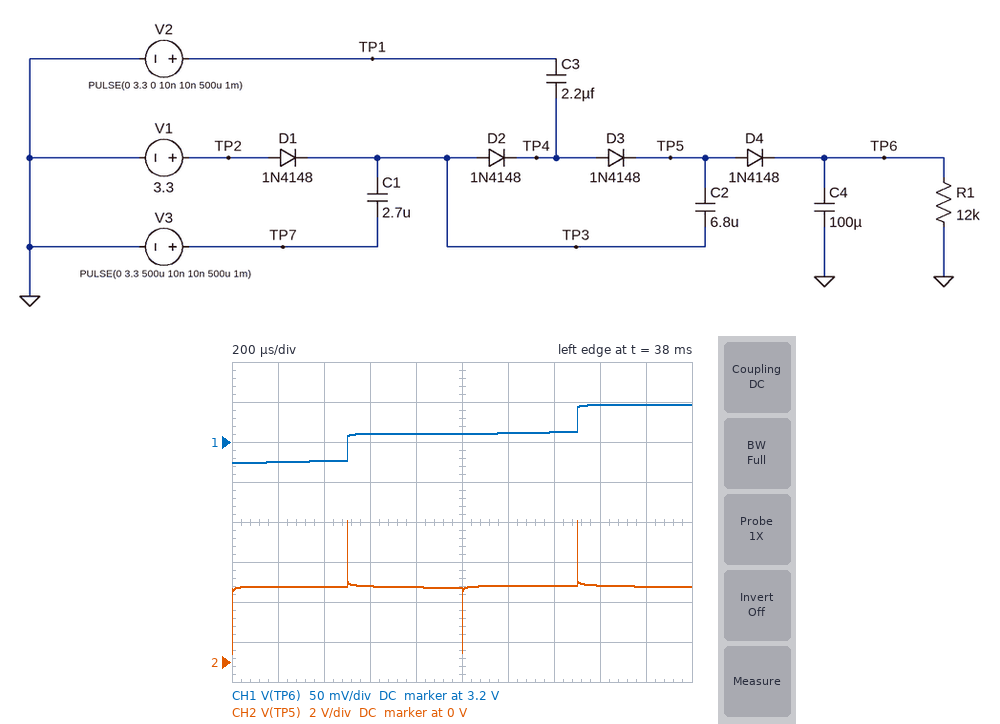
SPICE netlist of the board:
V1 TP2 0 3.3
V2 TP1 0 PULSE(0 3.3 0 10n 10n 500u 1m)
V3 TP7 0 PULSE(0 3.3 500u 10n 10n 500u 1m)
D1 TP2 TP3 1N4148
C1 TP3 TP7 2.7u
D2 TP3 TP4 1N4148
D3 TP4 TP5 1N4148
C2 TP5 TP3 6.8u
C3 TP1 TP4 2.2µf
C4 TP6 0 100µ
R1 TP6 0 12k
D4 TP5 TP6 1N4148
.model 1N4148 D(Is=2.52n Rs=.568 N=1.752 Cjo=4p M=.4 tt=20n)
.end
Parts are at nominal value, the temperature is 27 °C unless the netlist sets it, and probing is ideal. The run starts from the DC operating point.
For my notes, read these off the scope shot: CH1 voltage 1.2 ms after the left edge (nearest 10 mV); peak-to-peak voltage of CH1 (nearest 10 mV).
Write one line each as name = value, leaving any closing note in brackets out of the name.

CH1 voltage 1.2 ms after the left edge = 3.21 V
peak-to-peak voltage of CH1 = 70 mV
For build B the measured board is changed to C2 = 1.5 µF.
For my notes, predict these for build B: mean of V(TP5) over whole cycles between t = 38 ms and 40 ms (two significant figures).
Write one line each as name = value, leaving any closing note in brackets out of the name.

mean of V(TP5) over whole cycles between t = 38 ms and 40 ms = 4.0 V
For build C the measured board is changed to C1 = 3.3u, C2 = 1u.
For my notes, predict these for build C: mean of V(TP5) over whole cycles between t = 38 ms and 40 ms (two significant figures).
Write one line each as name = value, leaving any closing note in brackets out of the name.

mean of V(TP5) over whole cycles between t = 38 ms and 40 ms = 4.2 V
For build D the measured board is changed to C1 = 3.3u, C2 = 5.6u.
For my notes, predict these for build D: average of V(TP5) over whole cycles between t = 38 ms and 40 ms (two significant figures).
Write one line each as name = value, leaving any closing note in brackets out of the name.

average of V(TP5) over whole cycles between t = 38 ms and 40 ms = 3.9 V
